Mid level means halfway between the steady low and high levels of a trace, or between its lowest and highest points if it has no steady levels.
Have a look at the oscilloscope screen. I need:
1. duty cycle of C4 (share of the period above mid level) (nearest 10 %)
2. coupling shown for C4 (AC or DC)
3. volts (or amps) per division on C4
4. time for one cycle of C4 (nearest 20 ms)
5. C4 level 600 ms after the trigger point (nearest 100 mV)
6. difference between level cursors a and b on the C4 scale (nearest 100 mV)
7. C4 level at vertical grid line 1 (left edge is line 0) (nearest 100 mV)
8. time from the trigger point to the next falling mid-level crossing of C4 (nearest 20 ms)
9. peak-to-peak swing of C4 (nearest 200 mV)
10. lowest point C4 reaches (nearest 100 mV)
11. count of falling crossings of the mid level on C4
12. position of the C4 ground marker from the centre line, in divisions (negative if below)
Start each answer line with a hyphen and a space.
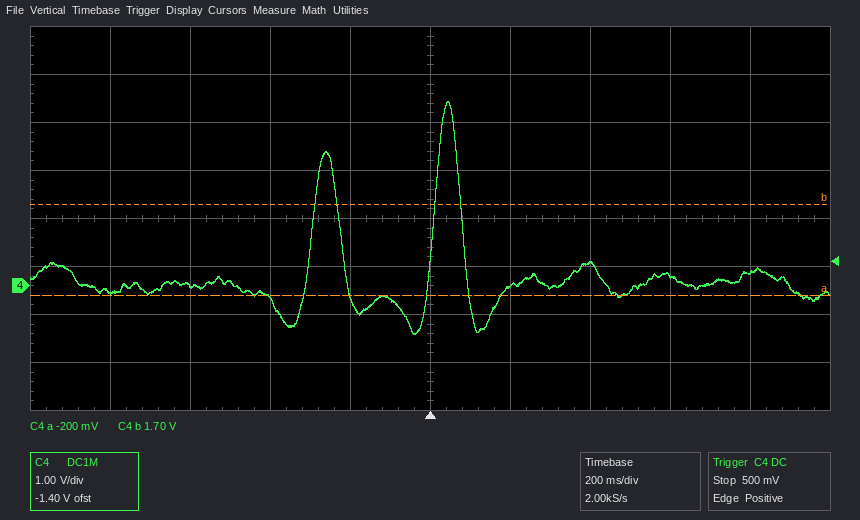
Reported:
- 20 %
- DC
- 1 V
- 300 ms
- 200 mV
- 1.9 V
- -100 mV
- 80 ms
- 4.8 V
- -1.0 V
- 2
- -1.4 div
